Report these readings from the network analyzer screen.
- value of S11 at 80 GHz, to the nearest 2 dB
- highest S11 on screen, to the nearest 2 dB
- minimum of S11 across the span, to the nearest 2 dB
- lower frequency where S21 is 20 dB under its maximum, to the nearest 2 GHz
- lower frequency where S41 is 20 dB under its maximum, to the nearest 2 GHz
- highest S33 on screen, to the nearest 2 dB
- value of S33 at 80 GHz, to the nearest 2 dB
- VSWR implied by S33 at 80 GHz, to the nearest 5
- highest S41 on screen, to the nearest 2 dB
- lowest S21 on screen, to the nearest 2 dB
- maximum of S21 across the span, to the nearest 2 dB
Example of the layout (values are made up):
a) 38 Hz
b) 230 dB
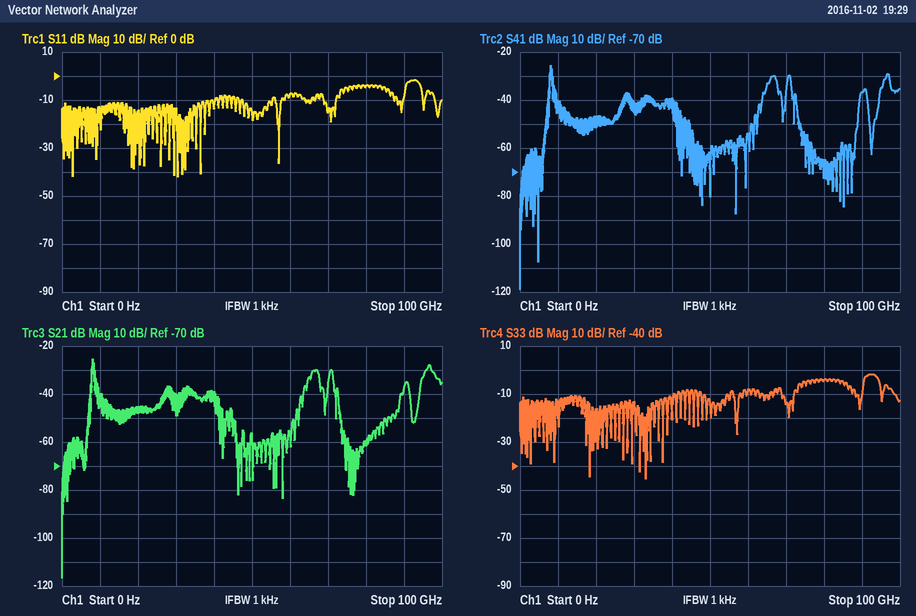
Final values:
a) -4 dB
b) -2 dB
c) -42 dB
d) 8 GHz
e) 8 GHz
f) -2 dB
g) -4 dB
h) 5
i) -26 dB
j) -116 dB
k) -26 dB
